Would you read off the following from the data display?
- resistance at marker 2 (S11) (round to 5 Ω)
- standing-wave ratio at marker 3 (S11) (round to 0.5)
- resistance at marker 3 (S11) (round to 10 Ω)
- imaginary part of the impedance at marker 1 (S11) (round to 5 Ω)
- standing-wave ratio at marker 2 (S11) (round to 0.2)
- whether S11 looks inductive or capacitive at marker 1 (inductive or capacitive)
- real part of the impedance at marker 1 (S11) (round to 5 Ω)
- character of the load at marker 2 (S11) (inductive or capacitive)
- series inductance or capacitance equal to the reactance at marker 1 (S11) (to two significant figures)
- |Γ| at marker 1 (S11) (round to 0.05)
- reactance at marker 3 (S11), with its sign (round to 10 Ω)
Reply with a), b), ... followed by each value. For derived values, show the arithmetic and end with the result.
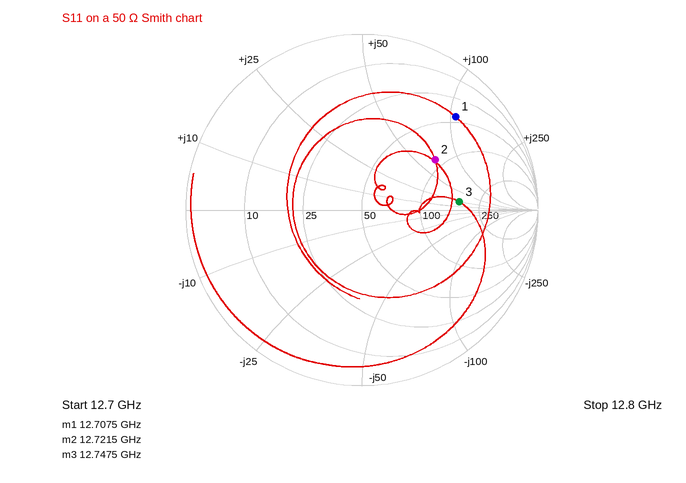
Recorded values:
a) 90 Ω
b) 3.5
c) 170 Ω
d) +105 Ω
e) 3.0
f) inductive
g) 45 Ω
h) inductive
i) L = 105 Ω/(2π × 12.7075 GHz) ≈ 1.3 nH
j) 0.75
k) +20 Ω
